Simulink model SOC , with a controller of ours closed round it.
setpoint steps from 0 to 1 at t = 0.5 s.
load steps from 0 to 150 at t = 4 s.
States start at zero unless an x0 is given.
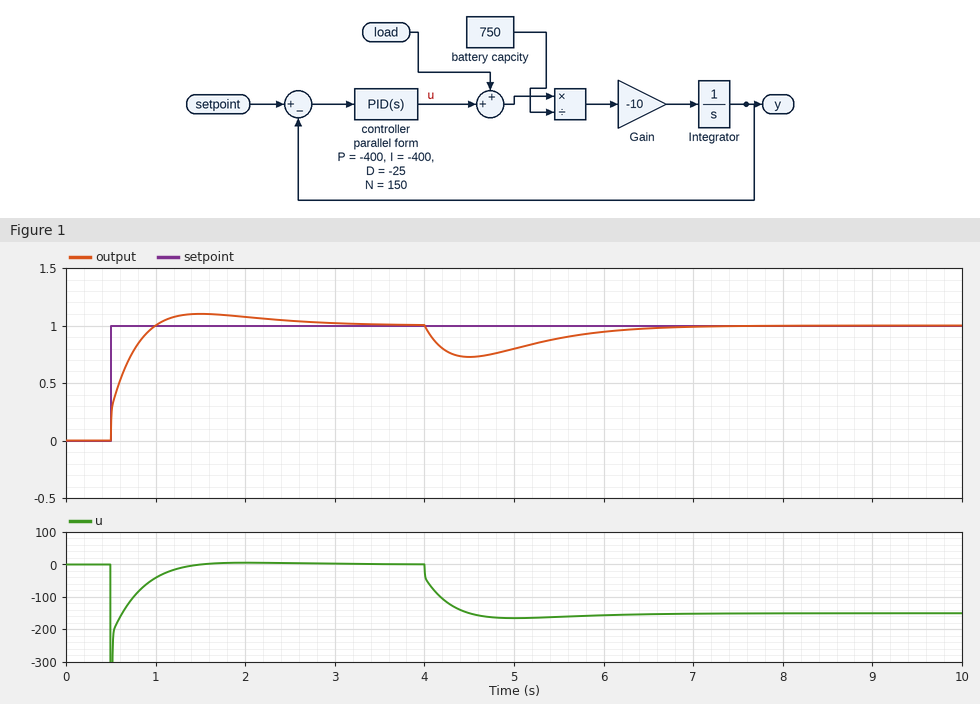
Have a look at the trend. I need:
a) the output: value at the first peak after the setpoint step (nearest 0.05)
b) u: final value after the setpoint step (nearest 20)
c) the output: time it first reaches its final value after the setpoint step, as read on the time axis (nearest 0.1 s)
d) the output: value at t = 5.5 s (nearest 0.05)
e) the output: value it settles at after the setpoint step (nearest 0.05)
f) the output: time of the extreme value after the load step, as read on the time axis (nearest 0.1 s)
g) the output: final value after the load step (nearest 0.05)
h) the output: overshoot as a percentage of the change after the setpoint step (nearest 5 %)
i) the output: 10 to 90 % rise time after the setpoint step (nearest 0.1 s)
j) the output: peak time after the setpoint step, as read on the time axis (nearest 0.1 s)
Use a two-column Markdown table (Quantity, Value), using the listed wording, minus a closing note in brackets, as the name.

| Quantity | Value |
|---|---|
| the output: value at the first peak after the setpoint step | 1.10 |
| u: final value after the setpoint step | 0 |
| the output: time it first reaches its final value after the setpoint step, as read on the time axis | 1.0 s |
| the output: value at t = 5.5 s | 0.90 |
| the output: value it settles at after the setpoint step | 1.00 |
| the output: time of the extreme value after the load step, as read on the time axis | 4.5 s |
| the output: final value after the load step | 1.00 |
| the output: overshoot as a percentage of the change after the setpoint step | 10 % |
| the output: 10 to 90 % rise time after the setpoint step | 0.4 s |
| the output: peak time after the setpoint step, as read on the time axis | 1.5 s |
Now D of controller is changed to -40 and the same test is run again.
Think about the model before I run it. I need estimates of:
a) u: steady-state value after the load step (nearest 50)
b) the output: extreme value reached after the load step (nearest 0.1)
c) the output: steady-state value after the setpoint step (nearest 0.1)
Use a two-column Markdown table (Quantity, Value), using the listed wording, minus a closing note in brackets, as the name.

| Quantity | Value |
|---|---|
| u: steady-state value after the load step | -150 |
| the output: extreme value reached after the load step | 0.7 |
| the output: steady-state value after the setpoint step | 1.0 |
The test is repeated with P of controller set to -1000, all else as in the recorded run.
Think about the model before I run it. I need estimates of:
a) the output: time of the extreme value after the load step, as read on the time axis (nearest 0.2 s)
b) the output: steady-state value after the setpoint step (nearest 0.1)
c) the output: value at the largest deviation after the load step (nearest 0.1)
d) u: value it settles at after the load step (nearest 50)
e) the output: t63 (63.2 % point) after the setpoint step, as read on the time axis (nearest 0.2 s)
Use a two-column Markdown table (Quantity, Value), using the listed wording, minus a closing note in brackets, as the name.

| Quantity | Value |
|---|---|
| the output: time of the extreme value after the load step, as read on the time axis | 4.4 s |
| the output: steady-state value after the setpoint step | 1.0 |
| the output: value at the largest deviation after the load step | 0.9 |
| u: value it settles at after the load step | -150 |
| the output: t63 (63.2 % point) after the setpoint step, as read on the time axis | 0.6 s |
